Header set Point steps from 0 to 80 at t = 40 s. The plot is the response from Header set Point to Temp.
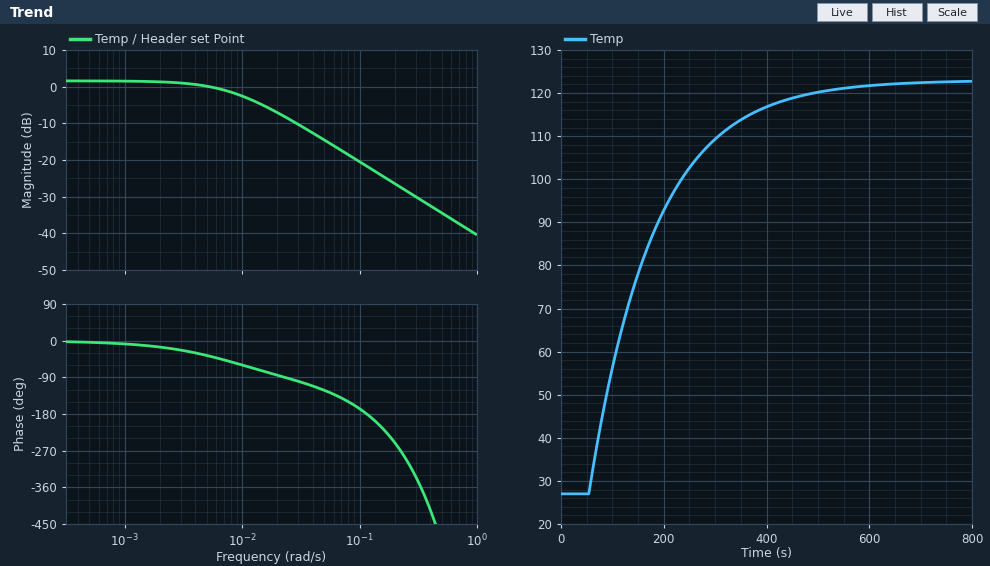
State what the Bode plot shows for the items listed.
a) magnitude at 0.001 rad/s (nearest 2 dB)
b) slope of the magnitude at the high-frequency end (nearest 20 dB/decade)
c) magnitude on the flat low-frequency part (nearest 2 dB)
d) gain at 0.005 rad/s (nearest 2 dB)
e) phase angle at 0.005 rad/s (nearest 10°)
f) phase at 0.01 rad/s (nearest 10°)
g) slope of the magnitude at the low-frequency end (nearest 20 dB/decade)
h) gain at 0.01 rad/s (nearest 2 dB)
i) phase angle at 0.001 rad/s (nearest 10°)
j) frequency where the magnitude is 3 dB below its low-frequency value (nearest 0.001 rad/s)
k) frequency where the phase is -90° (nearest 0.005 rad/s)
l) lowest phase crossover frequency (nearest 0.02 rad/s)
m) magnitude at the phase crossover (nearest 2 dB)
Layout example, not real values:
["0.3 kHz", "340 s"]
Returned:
["2 dB", "-20 dB/decade", "2 dB", "0 dB", "-40°", "-60°", "0 dB/decade", "-2 dB", "-10°", "0.008 rad/s", "0.025 rad/s", "0.12 rad/s", "-22 dB"]
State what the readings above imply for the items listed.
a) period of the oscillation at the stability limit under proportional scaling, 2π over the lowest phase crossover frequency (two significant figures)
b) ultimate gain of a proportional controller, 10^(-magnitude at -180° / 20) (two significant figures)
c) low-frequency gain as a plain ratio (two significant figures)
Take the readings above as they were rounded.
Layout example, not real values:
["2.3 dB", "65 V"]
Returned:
["52 s", "13", "1.3"]
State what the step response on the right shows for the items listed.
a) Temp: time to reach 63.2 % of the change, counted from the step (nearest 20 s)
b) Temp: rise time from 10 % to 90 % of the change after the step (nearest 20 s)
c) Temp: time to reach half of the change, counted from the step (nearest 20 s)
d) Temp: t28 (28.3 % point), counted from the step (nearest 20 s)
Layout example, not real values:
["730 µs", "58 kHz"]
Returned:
["140 s", "280 s", "100 s", "60 s"]
